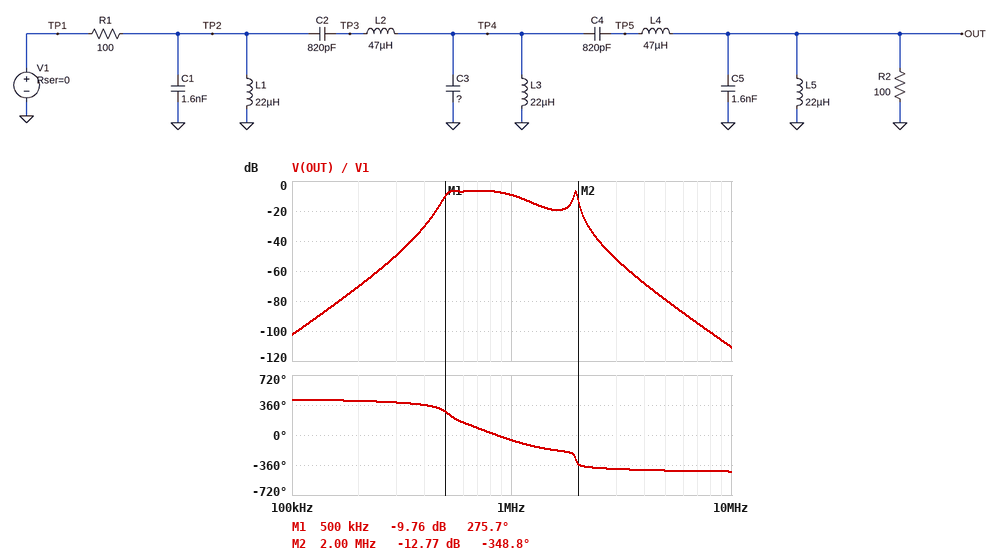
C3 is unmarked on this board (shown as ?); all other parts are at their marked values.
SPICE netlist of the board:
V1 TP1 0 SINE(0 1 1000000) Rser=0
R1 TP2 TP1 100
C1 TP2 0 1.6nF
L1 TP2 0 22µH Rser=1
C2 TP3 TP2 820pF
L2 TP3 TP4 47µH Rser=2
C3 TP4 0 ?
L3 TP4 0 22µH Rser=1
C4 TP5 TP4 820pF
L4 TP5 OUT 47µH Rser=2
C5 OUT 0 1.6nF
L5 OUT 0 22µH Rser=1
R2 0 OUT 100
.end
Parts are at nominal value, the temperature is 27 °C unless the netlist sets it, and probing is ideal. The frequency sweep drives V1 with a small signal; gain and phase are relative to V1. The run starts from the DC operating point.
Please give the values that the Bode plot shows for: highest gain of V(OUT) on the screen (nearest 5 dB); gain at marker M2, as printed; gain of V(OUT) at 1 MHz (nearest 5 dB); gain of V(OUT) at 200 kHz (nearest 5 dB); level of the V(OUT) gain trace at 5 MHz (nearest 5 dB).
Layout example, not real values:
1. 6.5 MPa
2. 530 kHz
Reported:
1. -5 dB
2. -12.77 dB
3. -10 dB
4. -70 dB
5. -80 dB
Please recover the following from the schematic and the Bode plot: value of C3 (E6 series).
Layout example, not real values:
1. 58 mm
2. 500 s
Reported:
1. 680 pF
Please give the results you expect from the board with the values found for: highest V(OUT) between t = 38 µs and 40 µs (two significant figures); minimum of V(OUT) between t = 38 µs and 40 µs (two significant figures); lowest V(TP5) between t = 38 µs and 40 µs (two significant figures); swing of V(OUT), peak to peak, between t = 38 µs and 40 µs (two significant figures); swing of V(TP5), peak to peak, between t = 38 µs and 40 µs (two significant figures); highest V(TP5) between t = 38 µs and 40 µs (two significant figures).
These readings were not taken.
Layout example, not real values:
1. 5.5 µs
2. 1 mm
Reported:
1. 340 mV
2. -340 mV
3. -1.0 V
4. 680 mV
5. 2.0 V
6. 1.0 V
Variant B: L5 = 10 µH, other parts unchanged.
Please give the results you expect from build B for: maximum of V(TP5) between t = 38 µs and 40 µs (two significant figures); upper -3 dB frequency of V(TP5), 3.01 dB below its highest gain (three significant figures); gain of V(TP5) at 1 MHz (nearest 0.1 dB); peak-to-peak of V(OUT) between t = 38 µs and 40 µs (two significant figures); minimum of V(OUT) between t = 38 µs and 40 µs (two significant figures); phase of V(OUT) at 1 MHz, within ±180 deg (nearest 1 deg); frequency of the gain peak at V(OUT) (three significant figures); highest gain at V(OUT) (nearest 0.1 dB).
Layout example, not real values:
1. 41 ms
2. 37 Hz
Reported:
1. 1.0 V
2. 1.99 MHz
3. 0.2 dB
4. 500 mV
5. -250 mV
6. -31 deg
7. 1.95 MHz
8. -7.0 dB
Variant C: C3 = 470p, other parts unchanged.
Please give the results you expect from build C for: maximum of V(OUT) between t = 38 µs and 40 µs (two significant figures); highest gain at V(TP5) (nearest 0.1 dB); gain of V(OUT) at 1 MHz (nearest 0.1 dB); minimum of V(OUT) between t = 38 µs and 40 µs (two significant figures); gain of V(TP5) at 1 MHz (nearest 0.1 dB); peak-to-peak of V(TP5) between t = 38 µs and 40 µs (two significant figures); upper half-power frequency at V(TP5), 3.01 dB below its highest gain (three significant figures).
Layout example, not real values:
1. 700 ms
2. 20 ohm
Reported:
1. 320 mV
2. 15.6 dB
3. -9.8 dB
4. -320 mV
5. -0.4 dB
6. 1.9 V
7. 2.32 MHz
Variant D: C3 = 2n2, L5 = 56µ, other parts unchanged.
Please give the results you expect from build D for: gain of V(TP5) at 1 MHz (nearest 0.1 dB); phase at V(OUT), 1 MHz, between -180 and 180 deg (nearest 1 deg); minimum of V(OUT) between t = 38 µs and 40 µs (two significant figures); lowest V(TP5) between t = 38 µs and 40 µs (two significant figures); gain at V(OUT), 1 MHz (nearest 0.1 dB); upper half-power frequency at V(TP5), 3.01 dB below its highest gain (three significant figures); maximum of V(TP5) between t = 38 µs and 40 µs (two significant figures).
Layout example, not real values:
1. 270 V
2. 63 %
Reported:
1. 3.0 dB
2. -108 deg
3. -450 mV
4. -1.4 V
5. -7.0 dB
6. 1.32 MHz
7. 1.4 V
